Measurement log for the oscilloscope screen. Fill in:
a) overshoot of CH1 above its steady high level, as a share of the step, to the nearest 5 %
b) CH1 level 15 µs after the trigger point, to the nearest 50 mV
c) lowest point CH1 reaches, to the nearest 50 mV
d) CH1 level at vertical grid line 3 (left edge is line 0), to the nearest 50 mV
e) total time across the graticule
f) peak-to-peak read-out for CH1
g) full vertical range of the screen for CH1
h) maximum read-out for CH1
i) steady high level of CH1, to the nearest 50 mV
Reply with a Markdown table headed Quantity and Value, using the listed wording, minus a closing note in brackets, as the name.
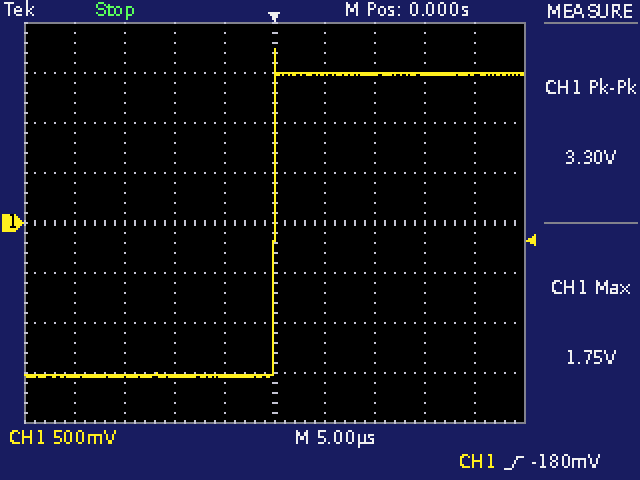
| Quantity | Value |
|---|---|
| overshoot of CH1 above its steady high level, as a share of the step, to the nearest 5 % | 10 % |
| CH1 level 15 µs after the trigger point, to the nearest 50 mV | 1.50 V |
| lowest point CH1 reaches, to the nearest 50 mV | -1.55 V |
| CH1 level at vertical grid line 3 (left edge is line 0), to the nearest 50 mV | -1.55 V |
| total time across the graticule | 50 µs |
| peak-to-peak read-out for CH1 | 3.30 V |
| full vertical range of the screen for CH1 | 4 V |
| maximum read-out for CH1 | 1.75 V |
| steady high level of CH1, to the nearest 50 mV | 1.50 V |
